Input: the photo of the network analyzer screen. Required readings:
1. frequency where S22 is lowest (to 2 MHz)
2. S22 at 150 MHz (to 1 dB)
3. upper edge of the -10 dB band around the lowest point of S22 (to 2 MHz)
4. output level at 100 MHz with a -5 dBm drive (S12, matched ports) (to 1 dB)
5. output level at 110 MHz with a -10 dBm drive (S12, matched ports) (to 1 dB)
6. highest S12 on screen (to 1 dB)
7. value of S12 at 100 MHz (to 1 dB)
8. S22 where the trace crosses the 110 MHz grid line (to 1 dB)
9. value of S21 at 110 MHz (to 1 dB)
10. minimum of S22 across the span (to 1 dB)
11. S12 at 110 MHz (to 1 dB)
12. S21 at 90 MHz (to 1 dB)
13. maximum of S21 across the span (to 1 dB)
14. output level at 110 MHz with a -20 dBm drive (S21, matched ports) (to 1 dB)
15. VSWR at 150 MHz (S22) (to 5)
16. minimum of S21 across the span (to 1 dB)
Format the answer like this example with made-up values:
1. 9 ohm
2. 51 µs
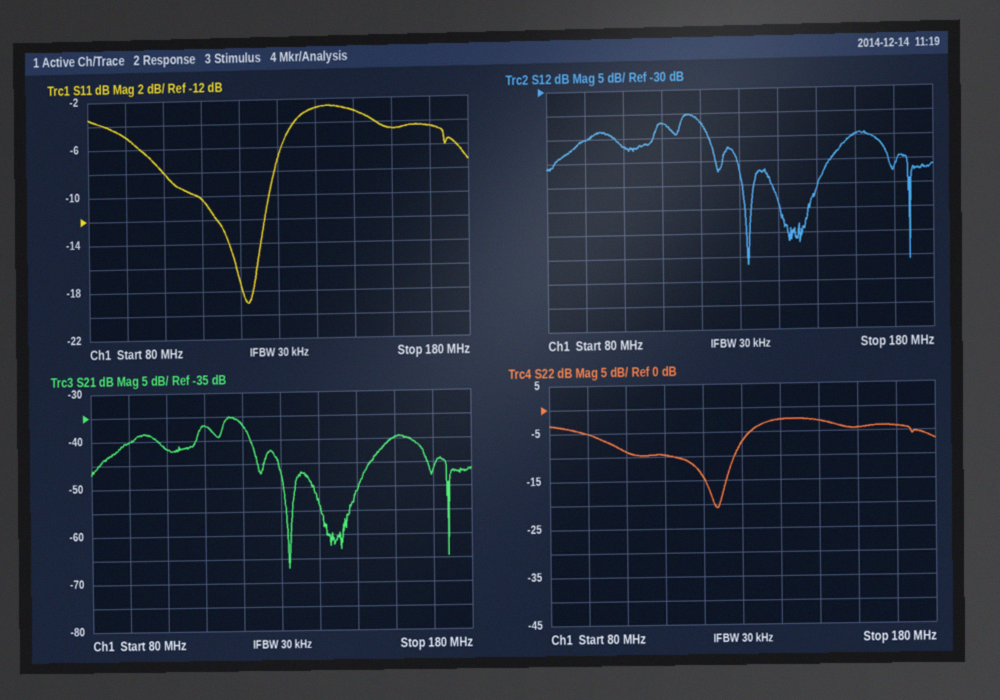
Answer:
1. 124 MHz
2. -3 dB
3. 128 MHz
4. -47 dBm
5. -47 dBm
6. -35 dB
7. -42 dB
8. -10 dB
9. -37 dB
10. -21 dB
11. -37 dB
12. -40 dB
13. -35 dB
14. -57 dBm
15. 5
16. -67 dB
